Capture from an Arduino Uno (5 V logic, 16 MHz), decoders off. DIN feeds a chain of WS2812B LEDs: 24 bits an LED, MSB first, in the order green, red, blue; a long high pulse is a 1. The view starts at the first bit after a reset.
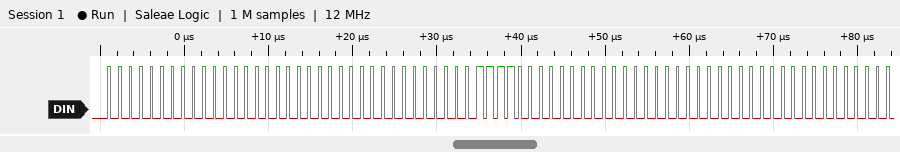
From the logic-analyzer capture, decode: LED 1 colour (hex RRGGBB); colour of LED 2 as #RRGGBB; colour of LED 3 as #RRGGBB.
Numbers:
#000000
#1E0000
#000000
